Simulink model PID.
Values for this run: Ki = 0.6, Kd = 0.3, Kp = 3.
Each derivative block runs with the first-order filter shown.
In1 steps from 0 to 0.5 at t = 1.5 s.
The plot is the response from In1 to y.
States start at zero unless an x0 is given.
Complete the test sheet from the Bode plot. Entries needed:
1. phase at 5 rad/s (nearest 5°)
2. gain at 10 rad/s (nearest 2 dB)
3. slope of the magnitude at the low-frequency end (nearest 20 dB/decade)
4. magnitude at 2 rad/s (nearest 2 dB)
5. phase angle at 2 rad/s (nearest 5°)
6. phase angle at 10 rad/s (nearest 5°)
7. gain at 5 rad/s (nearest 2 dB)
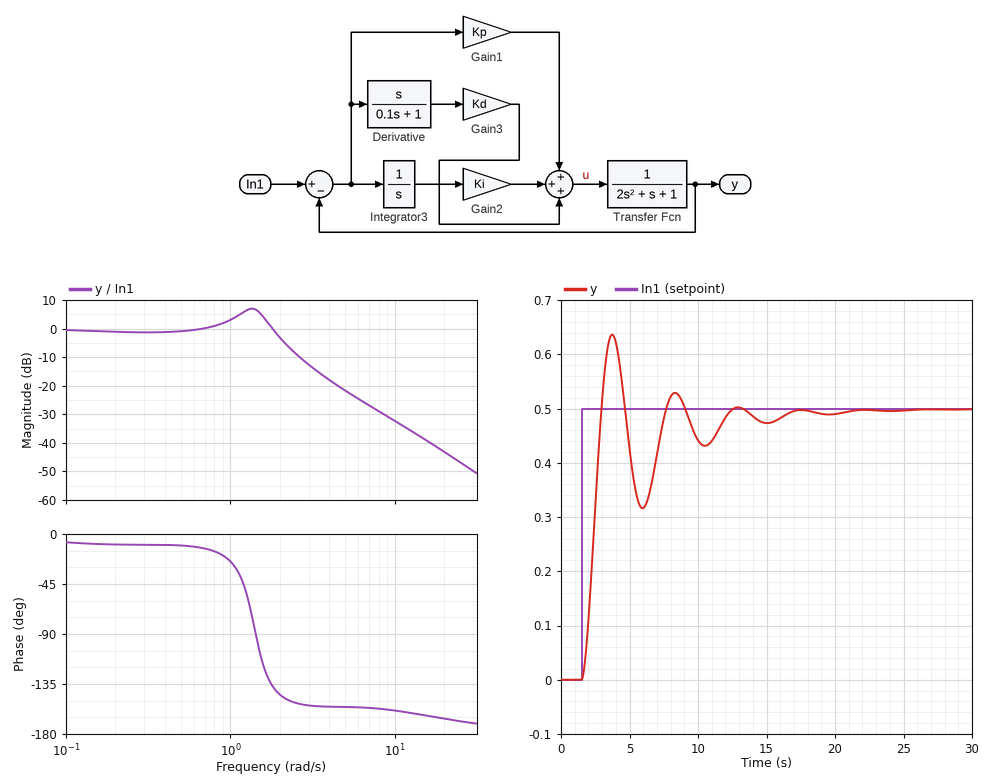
-155°
-32 dB
0 dB/decade
-4 dB
-145°
-160°
-22 dB
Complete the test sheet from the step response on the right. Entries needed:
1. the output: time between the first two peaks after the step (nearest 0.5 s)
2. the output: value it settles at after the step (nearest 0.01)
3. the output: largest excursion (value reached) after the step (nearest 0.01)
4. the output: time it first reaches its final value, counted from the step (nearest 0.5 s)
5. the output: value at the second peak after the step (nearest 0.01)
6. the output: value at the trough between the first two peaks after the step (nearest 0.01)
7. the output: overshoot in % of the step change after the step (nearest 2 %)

4.5 s
0.50
0.64
1.5 s
0.53
0.32
28 %
